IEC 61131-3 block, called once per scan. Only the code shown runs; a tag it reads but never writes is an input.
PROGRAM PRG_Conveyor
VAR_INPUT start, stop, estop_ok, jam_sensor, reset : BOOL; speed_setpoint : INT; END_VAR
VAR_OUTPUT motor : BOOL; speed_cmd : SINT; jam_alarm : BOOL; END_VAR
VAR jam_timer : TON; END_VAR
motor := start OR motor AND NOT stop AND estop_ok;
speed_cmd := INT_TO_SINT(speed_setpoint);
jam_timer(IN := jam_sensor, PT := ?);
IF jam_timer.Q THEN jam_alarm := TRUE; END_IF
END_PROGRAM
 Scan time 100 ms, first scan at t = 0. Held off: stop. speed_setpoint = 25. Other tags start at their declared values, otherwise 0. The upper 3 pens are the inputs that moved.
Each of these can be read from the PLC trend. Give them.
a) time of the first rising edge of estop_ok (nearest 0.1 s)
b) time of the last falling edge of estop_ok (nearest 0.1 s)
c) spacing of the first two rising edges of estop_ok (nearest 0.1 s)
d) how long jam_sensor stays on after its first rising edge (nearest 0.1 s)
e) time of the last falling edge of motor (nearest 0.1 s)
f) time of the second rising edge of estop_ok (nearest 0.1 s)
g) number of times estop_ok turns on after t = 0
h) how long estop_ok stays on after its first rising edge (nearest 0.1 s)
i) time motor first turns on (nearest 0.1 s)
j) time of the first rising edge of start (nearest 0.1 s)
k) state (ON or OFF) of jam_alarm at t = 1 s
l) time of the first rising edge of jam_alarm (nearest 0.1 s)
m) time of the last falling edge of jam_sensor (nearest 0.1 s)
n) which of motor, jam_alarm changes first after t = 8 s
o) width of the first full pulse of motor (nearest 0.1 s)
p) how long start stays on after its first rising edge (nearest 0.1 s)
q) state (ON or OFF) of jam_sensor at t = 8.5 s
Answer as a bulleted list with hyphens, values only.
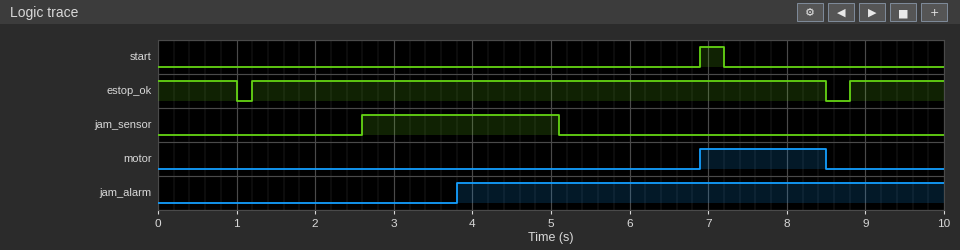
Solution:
- 1.2 s
- 8.5 s
- 7.6 s
- 2.5 s
- 8.5 s
- 8.8 s
- 2
- 7.3 s
- 6.9 s
- 6.9 s
- OFF
- 3.8 s
- 5.1 s
- motor
- 1.6 s
- 0.3 s
- OFF
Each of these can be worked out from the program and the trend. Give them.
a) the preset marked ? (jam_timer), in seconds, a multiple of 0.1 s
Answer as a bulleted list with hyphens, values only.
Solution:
- 1.2 s
